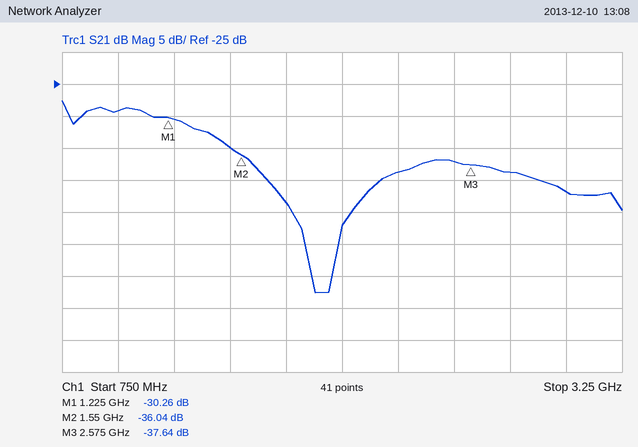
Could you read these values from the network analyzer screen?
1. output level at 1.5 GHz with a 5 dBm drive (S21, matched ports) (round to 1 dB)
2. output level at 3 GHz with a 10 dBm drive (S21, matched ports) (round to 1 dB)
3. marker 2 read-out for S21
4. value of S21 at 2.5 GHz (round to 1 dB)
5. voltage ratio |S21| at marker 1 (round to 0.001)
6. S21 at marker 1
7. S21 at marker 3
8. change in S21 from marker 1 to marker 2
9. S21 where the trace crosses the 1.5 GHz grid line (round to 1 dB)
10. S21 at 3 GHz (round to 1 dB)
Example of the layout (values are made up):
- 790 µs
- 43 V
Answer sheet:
- -30 dBm
- -32 dBm
- -36.04 dB
- -37 dB
- 0.031
- -30.26 dB
- -37.64 dB
- -5.78 dB
- -35 dB
- -42 dB
